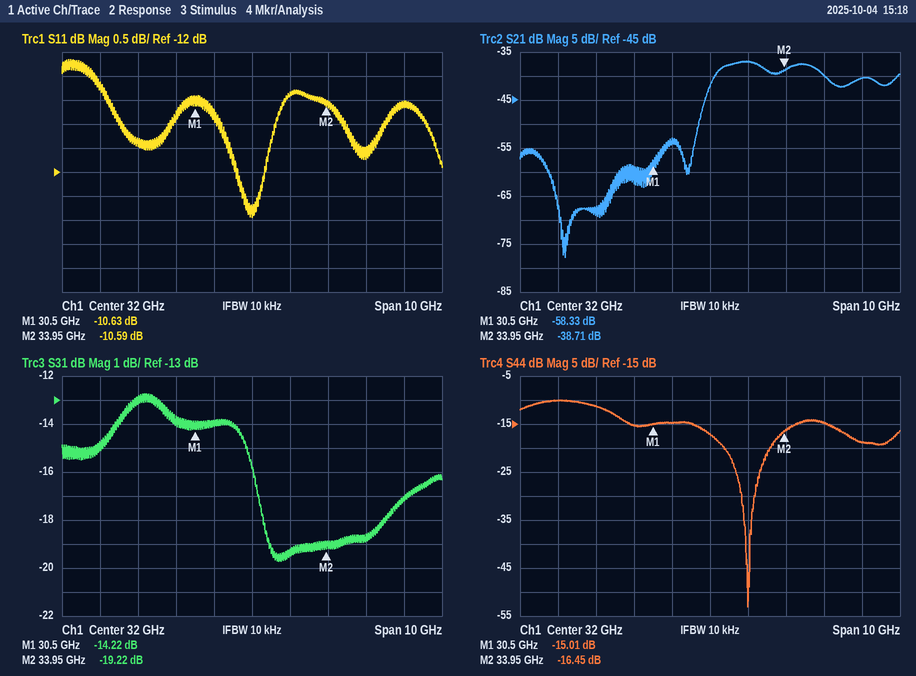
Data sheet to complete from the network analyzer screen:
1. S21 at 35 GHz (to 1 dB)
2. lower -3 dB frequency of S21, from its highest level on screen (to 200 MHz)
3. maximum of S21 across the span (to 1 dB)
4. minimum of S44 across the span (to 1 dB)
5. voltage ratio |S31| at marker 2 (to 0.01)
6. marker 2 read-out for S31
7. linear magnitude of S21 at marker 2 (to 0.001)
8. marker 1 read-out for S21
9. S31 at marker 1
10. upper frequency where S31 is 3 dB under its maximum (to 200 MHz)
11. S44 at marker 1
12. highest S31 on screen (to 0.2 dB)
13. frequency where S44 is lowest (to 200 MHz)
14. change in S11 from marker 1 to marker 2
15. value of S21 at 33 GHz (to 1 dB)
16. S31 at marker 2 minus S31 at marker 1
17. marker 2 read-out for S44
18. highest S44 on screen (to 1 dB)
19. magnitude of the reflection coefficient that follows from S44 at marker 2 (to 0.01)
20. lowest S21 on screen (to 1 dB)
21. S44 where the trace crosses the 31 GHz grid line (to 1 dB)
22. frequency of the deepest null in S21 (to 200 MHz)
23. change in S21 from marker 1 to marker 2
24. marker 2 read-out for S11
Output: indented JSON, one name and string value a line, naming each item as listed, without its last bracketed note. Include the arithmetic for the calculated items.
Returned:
{
  "S21 at 35 GHz": "-40 dB",
  "lower -3 dB frequency of S21, from its highest level on screen": "32.2 GHz",
  "maximum of S21 across the span": "-37 dB",
  "minimum of S44 across the span": "-53 dB",
  "voltage ratio |S31| at marker 2": "10^(-19.22/20) ≈ 0.11",
  "marker 2 read-out for S31": "-19.22 dB",
  "linear magnitude of S21 at marker 2": "10^(-38.71/20) ≈ 0.012",
  "marker 1 read-out for S21": "-58.33 dB",
  "S31 at marker 1": "-14.22 dB",
  "upper frequency where S31 is 3 dB under its maximum": "32.0 GHz",
  "S44 at marker 1": "-15.01 dB",
  "highest S31 on screen": "-12.8 dB",
  "frequency where S44 is lowest": "33.0 GHz",
  "change in S11 from marker 1 to marker 2": "-10.59 − (-10.63) = 0.04 dB",
  "value of S21 at 33 GHz": "-37 dB",
  "S31 at marker 2 minus S31 at marker 1": "-19.22 − (-14.22) = -5.00 dB",
  "marker 2 read-out for S44": "-16.45 dB",
  "highest S44 on screen": "-10 dB",
  "magnitude of the reflection coefficient that follows from S44 at marker 2": "10^(-16.45/20) ≈ 0.15",
  "lowest S21 on screen": "-78 dB",
  "S44 where the trace crosses the 31 GHz grid line": "-15 dB",
  "frequency of the deepest null in S21": "28.2 GHz",
  "change in S21 from marker 1 to marker 2": "-38.71 − (-58.33) = 19.62 dB",
  "marker 2 read-out for S11": "-10.59 dB"
}
